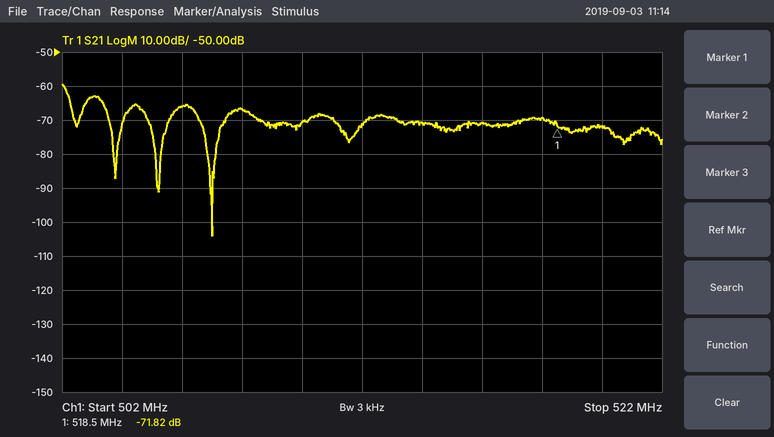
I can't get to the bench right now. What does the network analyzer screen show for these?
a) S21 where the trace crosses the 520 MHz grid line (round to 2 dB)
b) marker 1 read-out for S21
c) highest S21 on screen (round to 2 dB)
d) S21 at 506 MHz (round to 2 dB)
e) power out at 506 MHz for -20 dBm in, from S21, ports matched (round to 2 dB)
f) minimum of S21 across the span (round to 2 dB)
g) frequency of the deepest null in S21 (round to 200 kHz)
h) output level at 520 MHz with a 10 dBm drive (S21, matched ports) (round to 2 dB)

-72 dB
-71.82 dB
-60 dB
-66 dB
-86 dBm
-104 dB
507.0 MHz
-62 dBm
